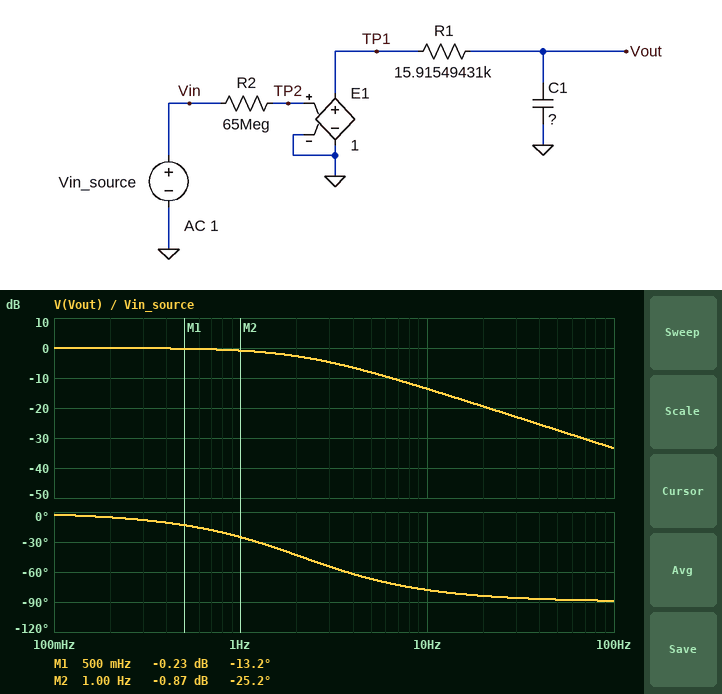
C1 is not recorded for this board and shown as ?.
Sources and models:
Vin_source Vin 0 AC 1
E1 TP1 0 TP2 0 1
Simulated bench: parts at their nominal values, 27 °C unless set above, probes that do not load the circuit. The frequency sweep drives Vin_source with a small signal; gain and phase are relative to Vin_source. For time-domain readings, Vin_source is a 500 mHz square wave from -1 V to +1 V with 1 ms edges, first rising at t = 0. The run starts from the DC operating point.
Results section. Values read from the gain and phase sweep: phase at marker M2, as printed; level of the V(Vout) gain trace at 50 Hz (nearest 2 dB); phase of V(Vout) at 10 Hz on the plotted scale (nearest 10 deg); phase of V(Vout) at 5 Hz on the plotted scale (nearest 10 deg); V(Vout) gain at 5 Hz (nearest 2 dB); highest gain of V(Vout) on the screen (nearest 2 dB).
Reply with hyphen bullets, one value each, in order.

- -25.2 deg
- -28 dB
- -80 deg
- -70 deg
- -8 dB
- 0 dB
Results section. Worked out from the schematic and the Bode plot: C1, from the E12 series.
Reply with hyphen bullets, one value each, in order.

- 4.7 µF
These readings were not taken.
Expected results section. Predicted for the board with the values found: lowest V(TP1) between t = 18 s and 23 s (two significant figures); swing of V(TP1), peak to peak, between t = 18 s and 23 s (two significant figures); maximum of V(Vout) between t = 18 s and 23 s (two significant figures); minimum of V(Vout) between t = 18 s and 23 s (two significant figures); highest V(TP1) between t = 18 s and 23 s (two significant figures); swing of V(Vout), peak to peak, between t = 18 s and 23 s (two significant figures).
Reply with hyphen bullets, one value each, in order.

- -1.0 V
- 2.0 V
- 1.0 V
- -1.0 V
- 1.0 V
- 2.0 V
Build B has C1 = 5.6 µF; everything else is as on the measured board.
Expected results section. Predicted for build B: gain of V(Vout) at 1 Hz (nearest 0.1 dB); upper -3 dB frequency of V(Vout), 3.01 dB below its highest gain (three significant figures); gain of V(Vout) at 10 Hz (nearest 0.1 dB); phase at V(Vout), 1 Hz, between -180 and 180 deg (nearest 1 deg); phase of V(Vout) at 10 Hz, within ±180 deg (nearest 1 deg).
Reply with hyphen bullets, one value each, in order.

- -1.2 dB
- 1.79 Hz
- -15.1 dB
- -29 deg
- -80 deg
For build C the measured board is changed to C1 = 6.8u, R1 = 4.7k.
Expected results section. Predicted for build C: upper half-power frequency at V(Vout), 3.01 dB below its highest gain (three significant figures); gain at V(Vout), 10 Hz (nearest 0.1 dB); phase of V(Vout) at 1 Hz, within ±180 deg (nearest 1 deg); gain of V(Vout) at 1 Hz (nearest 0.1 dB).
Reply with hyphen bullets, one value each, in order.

- 4.98 Hz
- -7.0 dB
- -11 deg
- -0.2 dB
